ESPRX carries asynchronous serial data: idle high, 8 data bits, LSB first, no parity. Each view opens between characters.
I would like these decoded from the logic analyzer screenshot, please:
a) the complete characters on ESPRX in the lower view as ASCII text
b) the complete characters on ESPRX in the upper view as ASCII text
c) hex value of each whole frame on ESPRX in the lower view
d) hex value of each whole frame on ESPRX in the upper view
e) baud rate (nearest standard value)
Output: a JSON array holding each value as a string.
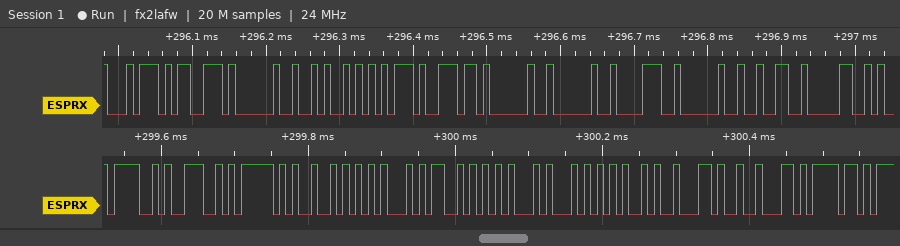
["\"ON_RESET),bo\"", "\"ts Jun  8 20\"", "4F, 4E, 5F, 52, 45, 53, 45, 54, 29, 2C, 62, 6F", "74, 73, 20, 4A, 75, 6E, 20, 20, 38, 20, 32, 30", "115200 baud"]
